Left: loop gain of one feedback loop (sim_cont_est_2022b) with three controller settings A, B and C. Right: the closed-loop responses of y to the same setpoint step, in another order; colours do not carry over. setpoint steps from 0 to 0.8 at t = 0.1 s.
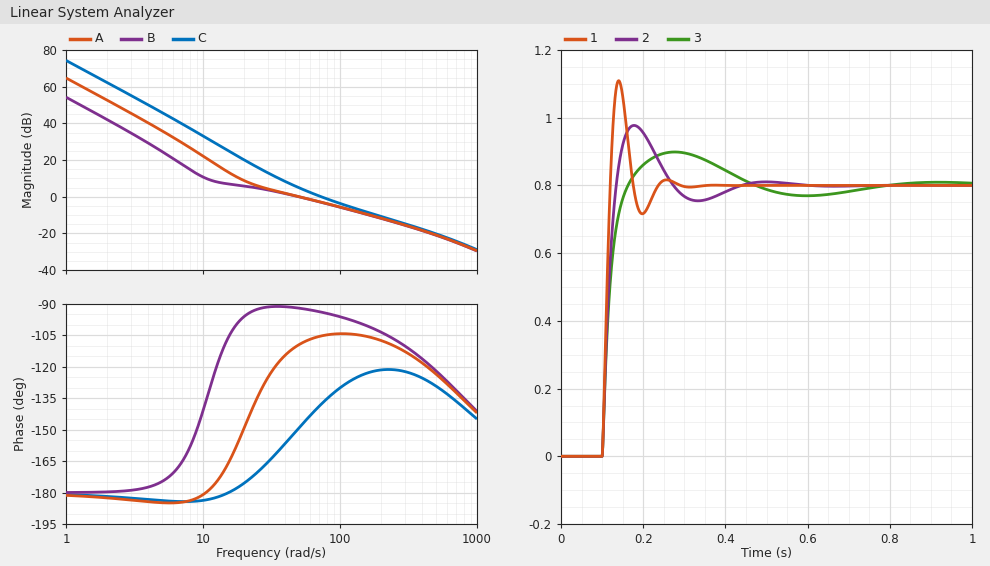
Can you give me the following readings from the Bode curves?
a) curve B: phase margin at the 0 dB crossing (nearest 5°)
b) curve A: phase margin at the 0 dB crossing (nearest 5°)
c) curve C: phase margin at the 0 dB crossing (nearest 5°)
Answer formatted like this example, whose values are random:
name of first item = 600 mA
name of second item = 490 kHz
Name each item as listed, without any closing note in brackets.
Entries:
curve B: phase margin at the 0 dB crossing = 90°
curve A: phase margin at the 0 dB crossing = 70°
curve C: phase margin at the 0 dB crossing = 40°
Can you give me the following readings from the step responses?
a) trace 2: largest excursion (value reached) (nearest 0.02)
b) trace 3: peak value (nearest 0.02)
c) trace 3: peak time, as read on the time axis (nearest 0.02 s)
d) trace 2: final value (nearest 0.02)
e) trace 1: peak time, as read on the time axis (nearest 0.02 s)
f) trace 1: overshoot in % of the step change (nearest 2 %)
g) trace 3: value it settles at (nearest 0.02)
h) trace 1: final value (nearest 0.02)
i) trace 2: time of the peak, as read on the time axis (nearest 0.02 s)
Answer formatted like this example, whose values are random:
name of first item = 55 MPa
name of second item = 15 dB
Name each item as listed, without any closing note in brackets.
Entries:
trace 2: largest excursion (value reached) = 0.98
trace 3: peak value = 0.90
trace 3: peak time, as read on the time axis = 0.28 s
trace 2: final value = 0.80
trace 1: peak time, as read on the time axis = 0.14 s
trace 1: overshoot in % of the step change = 38 %
trace 3: value it settles at = 0.80
trace 1: final value = 0.80
trace 2: time of the peak, as read on the time axis = 0.18 s
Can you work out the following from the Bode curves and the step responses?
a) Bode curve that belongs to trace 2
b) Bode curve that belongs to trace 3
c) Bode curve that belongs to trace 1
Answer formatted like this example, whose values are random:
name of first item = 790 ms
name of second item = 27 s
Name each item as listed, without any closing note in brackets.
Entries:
Bode curve that belongs to trace 2 = A
Bode curve that belongs to trace 3 = B
Bode curve that belongs to trace 1 = C
